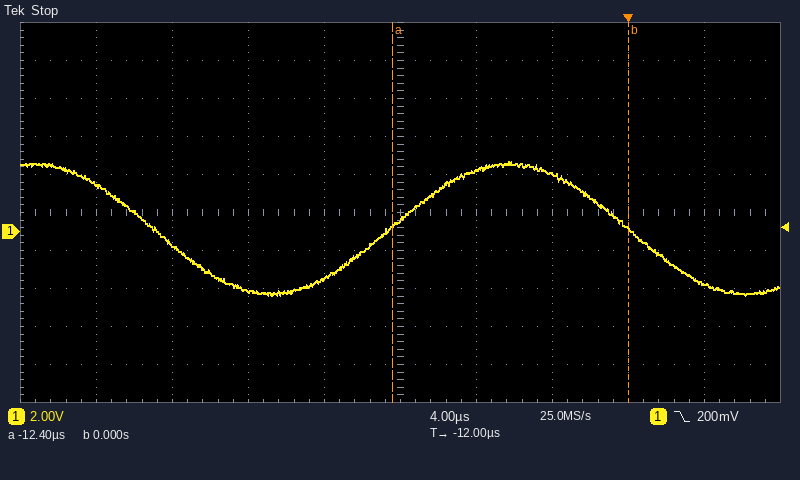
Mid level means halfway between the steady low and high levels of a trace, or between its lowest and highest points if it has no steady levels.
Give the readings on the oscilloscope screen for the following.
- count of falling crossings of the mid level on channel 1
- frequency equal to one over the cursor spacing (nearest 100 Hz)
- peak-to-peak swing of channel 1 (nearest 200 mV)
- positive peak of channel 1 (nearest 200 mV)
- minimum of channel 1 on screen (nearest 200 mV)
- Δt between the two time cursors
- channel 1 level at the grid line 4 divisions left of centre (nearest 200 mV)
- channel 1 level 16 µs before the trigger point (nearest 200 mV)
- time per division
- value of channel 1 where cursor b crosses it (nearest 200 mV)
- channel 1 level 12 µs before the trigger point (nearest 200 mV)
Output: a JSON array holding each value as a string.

["2", "80.6 kHz", "7.0 V", "3.6 V", "-3.4 V", "12.4 µs", "2.4 V", "-2.4 V", "4 µs", "200 mV", "600 mV"]
